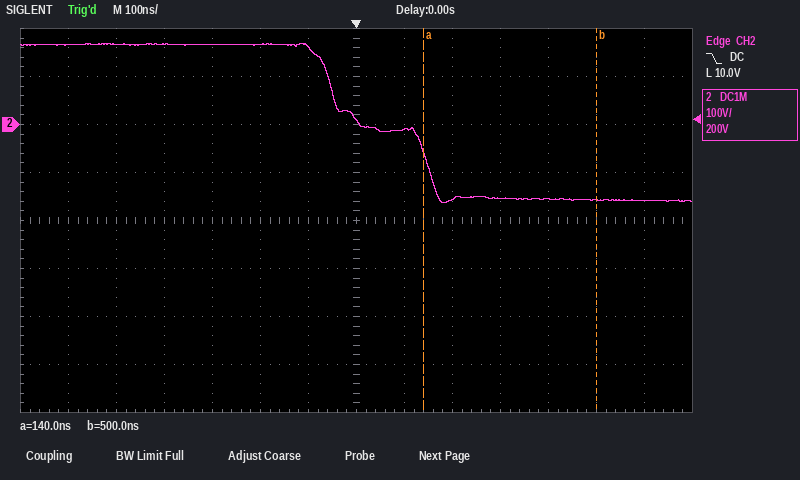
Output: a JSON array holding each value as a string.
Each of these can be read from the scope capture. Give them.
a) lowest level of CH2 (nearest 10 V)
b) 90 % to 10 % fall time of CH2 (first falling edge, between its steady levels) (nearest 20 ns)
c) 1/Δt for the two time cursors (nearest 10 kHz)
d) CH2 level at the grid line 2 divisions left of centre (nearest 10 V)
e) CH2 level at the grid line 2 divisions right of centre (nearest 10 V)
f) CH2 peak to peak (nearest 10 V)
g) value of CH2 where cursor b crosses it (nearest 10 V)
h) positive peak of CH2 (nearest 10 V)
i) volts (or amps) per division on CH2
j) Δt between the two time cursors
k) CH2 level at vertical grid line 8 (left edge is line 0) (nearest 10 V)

["-160 V", "240 ns", "2.78 MHz", "170 V", "-160 V", "330 V", "-160 V", "170 V", "100 V", "360 ns", "-10 V"]
